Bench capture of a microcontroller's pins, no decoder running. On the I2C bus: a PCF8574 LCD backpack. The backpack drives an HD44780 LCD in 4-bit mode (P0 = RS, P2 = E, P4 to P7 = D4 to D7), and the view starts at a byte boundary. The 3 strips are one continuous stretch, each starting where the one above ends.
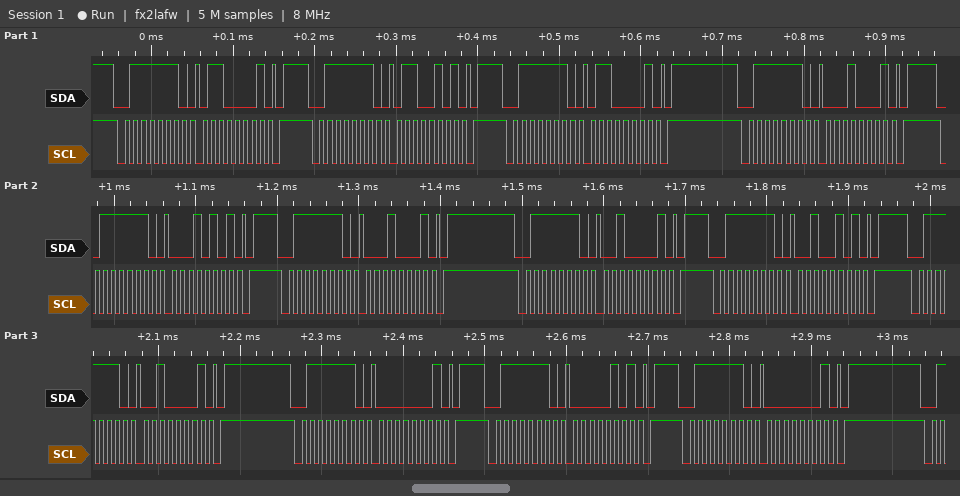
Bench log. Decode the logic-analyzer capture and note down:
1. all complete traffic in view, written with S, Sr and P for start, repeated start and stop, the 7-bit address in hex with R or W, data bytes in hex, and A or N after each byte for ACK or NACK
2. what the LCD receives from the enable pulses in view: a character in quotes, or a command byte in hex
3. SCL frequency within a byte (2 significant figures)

S 3FW A 61 A P S 3FW A 65 A P S 3FW A 61 A P S 3FW A 11 A P S 3FW A 15 A P S 3FW A 11 A P S 3FW A 21 A P S 3FW A 25 A P S 3FW A 21 A P S 3FW A 01 A P S 3FW A 05 A P S 3FW A 01 A P
'a' ' '
100 kHz
